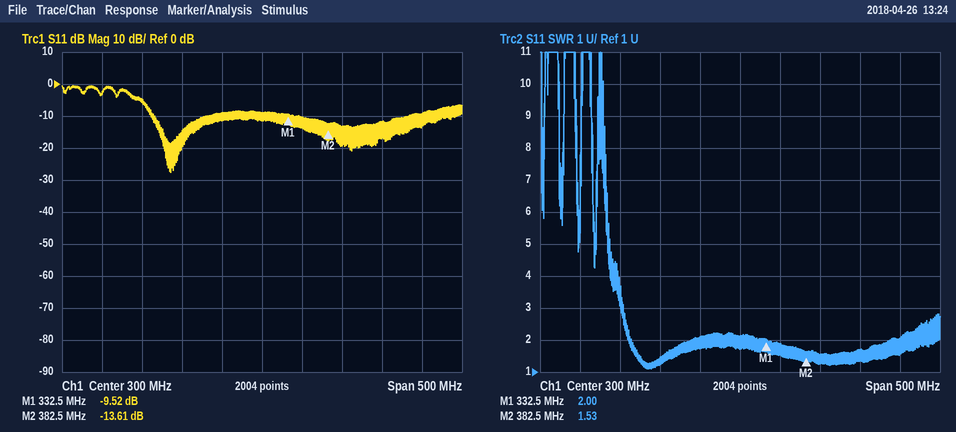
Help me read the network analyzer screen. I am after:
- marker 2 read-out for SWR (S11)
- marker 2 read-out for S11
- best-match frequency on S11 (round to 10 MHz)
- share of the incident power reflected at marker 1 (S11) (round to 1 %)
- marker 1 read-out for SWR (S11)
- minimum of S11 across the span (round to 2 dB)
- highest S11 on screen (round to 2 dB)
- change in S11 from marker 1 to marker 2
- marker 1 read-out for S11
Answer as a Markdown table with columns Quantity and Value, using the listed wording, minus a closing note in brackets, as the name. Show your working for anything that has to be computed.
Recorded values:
| Quantity | Value |
|---|---|
| marker 2 read-out for SWR | 1.53 |
| marker 2 read-out for S11 | -13.61 dB |
| best-match frequency on S11 | 190 MHz |
| share of the incident power reflected at marker 1 (S11) | 10^(-9.52/10) ≈ 11 % |
| marker 1 read-out for SWR | 2.00 |
| minimum of S11 across the span | -28 dB |
| highest S11 on screen | 0 dB |
| change in S11 from marker 1 to marker 2 | -13.61 − (-9.52) = -4.09 dB |
| marker 1 read-out for S11 | -9.52 dB |
